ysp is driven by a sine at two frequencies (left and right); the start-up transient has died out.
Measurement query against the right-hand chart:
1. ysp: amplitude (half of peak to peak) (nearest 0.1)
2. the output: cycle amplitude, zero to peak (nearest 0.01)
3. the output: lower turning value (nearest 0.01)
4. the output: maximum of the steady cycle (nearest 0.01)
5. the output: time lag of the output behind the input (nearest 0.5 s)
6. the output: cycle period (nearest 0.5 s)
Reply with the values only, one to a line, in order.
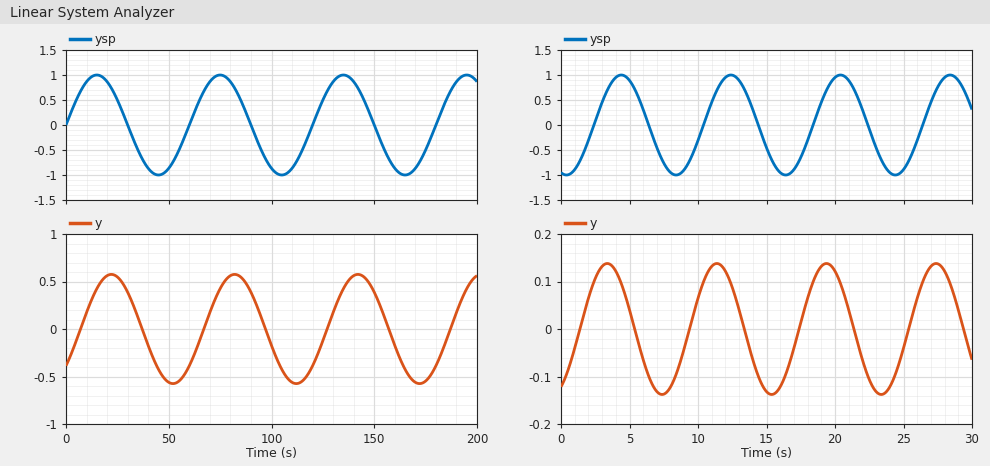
1.0
0.14
-0.14
0.14
7.0 s
8.0 s
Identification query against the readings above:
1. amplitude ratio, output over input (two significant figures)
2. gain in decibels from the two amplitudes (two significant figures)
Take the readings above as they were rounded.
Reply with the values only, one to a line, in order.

0.14
-17 dB
